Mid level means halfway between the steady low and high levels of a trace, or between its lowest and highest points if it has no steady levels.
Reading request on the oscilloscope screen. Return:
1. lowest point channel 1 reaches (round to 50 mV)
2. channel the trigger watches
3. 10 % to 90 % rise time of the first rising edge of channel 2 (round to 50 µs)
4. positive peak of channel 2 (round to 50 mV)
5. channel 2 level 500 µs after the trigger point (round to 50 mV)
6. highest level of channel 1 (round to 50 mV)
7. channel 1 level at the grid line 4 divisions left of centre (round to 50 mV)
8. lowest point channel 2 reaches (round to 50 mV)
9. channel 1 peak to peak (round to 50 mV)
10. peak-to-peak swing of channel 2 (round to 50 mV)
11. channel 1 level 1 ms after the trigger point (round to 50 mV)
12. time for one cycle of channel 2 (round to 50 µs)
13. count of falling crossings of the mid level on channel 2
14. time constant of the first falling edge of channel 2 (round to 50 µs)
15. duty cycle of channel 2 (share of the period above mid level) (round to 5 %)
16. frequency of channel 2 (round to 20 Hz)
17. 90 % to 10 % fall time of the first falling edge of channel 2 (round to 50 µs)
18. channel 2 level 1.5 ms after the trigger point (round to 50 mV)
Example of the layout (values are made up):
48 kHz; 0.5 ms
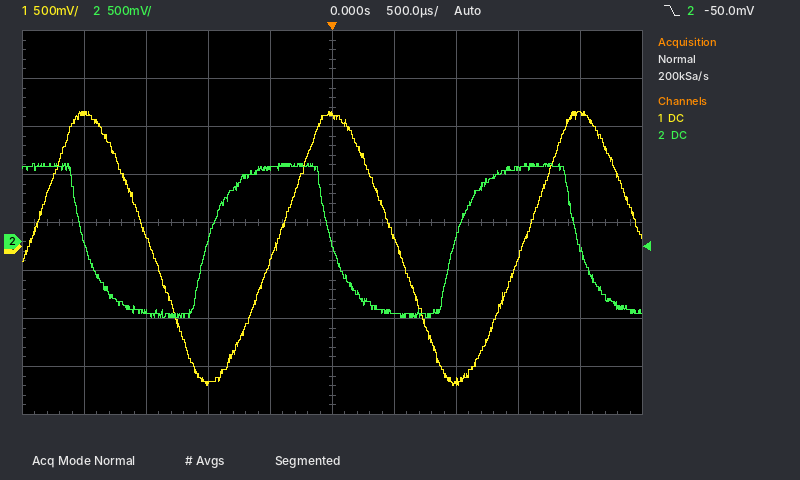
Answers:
-1.45 V; channel 2; 350 µs; 800 mV; -750 mV; 1.40 V; 1.40 V; -800 mV; 2.85 V; 1.60 V; -1.40 V; 2.00 ms; 3; 150 µs; 50 %; 500 Hz; 350 µs; 750 mV
